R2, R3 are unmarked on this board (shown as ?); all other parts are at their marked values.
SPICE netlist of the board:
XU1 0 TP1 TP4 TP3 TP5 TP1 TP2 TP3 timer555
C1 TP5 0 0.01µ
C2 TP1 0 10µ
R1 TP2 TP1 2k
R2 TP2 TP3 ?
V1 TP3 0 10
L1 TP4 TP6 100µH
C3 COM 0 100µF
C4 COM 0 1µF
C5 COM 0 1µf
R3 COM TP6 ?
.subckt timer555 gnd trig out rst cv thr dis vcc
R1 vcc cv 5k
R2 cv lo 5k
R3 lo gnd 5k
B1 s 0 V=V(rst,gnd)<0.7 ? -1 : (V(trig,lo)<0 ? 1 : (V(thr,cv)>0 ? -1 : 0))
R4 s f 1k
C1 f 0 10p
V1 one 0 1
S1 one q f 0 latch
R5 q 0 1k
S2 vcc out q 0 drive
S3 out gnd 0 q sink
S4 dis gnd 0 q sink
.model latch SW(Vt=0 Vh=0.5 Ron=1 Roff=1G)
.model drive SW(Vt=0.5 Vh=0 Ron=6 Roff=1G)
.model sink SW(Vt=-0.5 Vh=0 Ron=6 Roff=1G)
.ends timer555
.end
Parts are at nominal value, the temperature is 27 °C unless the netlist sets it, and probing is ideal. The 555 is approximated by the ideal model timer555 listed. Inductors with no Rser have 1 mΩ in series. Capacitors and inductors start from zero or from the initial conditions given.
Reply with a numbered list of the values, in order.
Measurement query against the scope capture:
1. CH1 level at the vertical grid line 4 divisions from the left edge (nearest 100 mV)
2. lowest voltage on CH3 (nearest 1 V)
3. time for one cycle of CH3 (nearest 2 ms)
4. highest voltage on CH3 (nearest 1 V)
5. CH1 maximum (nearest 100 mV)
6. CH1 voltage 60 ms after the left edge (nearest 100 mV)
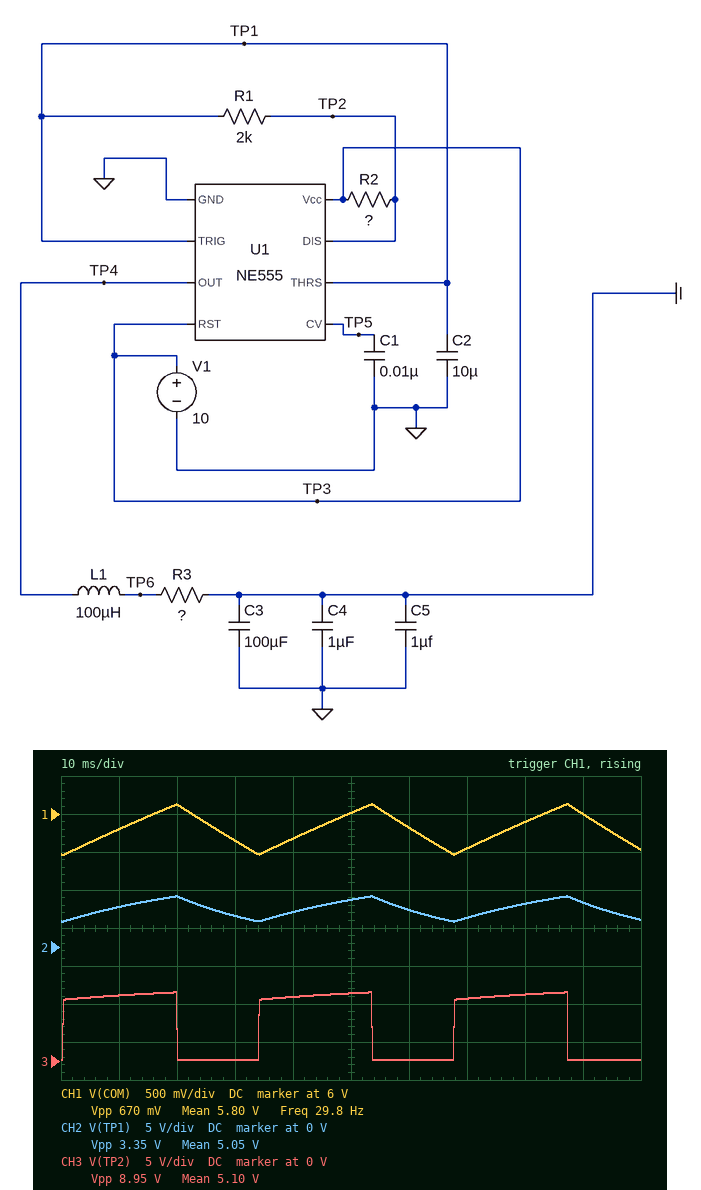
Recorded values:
1. 5.7 V
2. 0 V
3. 34 ms
4. 9 V
5. 6.1 V
6. 5.8 V
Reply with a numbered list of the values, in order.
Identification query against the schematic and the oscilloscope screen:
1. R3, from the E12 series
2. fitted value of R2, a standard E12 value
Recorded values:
1. 1.2 kΩ
2. 820 Ω
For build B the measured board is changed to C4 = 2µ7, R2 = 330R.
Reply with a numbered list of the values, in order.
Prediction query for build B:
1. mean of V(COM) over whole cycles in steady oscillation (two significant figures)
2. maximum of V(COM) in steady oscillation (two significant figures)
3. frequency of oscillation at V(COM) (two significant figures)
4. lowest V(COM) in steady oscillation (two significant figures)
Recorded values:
1. 5.3 V
2. 5.6 V
3. 33 Hz
4. 5.0 V
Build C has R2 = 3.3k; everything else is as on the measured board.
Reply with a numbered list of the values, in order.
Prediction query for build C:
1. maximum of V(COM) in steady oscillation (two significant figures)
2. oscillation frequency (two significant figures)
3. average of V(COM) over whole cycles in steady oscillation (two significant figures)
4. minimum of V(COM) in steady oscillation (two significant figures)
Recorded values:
1. 7.6 V
2. 20 Hz
3. 7.2 V
4. 6.8 V
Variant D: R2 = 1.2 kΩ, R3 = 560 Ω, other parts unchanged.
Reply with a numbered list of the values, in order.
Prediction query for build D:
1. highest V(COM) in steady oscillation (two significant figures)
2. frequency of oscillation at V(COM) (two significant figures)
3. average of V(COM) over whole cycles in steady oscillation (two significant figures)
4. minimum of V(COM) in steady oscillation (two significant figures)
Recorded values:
1. 6.8 V
2. 28 Hz
3. 6.1 V
4. 5.4 V
